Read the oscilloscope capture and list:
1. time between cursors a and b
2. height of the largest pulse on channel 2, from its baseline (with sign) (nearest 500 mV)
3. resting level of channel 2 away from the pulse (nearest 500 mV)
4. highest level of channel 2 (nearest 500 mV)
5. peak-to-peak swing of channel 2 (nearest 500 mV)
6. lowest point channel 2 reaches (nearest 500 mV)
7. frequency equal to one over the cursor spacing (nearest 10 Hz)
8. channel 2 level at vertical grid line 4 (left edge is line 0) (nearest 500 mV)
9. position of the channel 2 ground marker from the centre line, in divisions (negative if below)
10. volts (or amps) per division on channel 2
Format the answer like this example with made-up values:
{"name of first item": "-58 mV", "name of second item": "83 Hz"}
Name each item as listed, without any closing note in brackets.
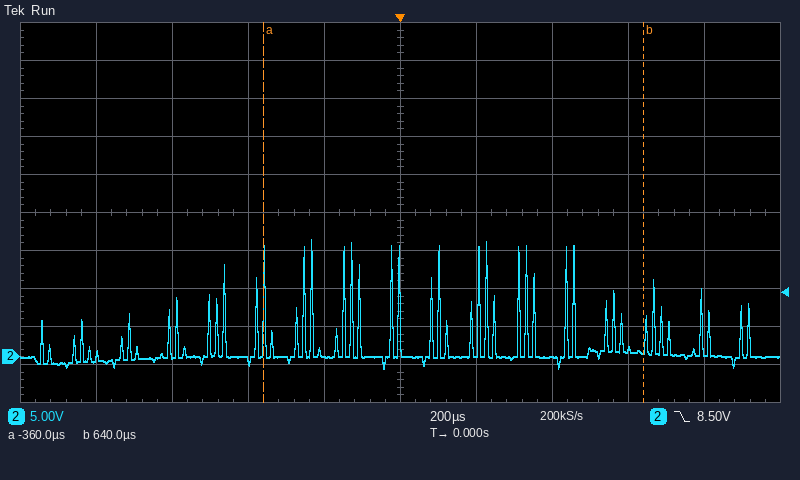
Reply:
{"time between cursors a and b": "1.00 ms", "height of the largest pulse on channel 2, from its baseline (with sign)": "+15.5 V", "resting level of channel 2 away from the pulse": "0.0 V", "highest level of channel 2": "15.5 V", "peak-to-peak swing of channel 2": "17.0 V", "lowest point channel 2 reaches": "-1.5 V", "frequency equal to one over the cursor spacing": "1.00 kHz", "channel 2 level at vertical grid line 4 (left edge is line 0)": "500 mV", "position of the channel 2 ground marker from the centre line, in divisions": "-3.8 div", "volts (or amps) per division on channel 2": "5 V"}
